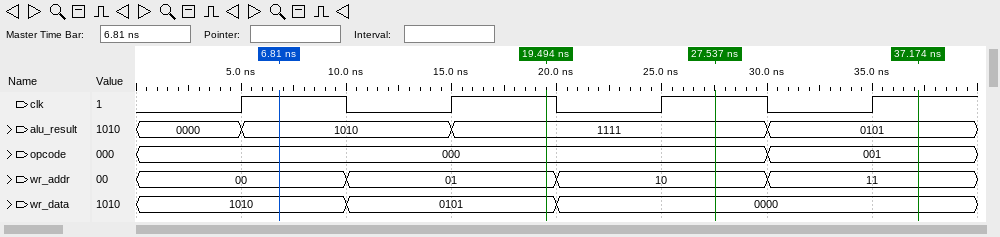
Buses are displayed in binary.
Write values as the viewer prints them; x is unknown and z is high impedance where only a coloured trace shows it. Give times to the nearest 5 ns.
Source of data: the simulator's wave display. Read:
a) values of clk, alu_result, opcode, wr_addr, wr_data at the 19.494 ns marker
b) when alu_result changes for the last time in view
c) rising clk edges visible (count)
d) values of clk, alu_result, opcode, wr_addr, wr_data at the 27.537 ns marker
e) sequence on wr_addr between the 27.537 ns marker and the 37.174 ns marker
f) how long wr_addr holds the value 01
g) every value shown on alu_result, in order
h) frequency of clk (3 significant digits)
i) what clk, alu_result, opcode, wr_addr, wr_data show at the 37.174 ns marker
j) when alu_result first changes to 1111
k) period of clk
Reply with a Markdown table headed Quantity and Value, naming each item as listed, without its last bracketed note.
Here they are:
| Quantity | Value |
|---|---|
| values of clk, alu_result, opcode, wr_addr, wr_data at the 19.494 ns marker | clk=1, alu_result=1111, opcode=000, wr_addr=01, wr_data=0101 |
| when alu_result changes for the last time in view | 30 ns |
| rising clk edges visible | 4 |
| values of clk, alu_result, opcode, wr_addr, wr_data at the 27.537 ns marker | clk=1, alu_result=1111, opcode=000, wr_addr=10, wr_data=0000 |
| sequence on wr_addr between the 27.537 ns marker and the 37.174 ns marker | 10, 11 |
| how long wr_addr holds the value 01 | 10 ns |
| every value shown on alu_result, in order | 0000, 1010, 1111, 0101 |
| frequency of clk | 100 MHz |
| what clk, alu_result, opcode, wr_addr, wr_data show at the 37.174 ns marker | clk=1, alu_result=0101, opcode=001, wr_addr=11, wr_data=0000 |
| when alu_result first changes to 1111 | 15 ns |
| period of clk | 10 ns |
